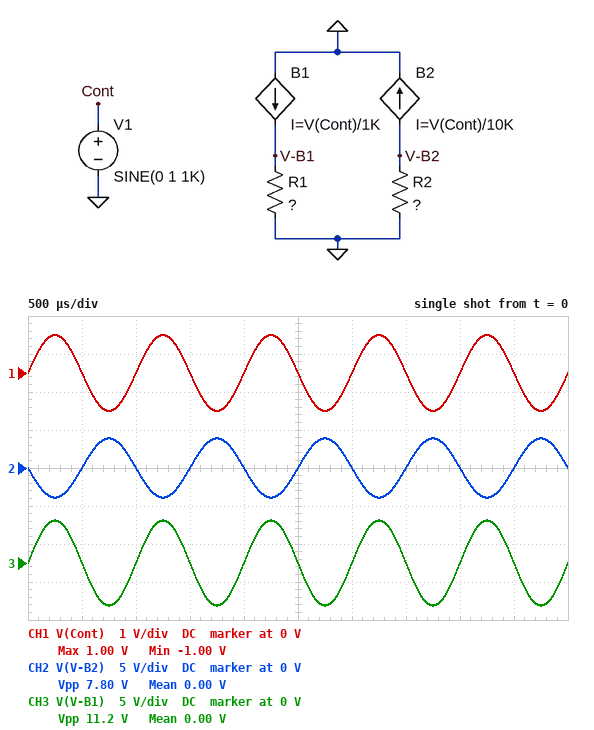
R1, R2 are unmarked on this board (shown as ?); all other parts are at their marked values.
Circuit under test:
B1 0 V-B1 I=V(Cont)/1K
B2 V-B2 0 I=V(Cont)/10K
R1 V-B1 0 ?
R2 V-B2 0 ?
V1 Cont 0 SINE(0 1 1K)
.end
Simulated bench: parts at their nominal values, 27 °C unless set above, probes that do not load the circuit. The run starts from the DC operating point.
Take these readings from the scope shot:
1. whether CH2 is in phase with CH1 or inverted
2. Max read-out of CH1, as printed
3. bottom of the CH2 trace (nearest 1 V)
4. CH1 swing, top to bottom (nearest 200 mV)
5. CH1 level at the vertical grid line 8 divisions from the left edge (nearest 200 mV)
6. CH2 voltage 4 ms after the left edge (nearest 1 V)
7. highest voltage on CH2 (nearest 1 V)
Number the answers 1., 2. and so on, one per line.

1. inverted
2. 1.00 V
3. -4 V
4. 2.0 V
5. 0 V
6. 0 V
7. 4 V
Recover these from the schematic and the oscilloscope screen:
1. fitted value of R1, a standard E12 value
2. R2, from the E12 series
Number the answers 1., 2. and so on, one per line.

1. 5.6 kΩ
2. 39 kΩ
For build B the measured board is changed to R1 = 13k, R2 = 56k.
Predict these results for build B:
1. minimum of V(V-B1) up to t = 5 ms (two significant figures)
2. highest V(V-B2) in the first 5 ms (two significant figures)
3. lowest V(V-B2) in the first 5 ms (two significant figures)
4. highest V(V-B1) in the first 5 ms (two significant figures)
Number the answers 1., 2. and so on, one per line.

1. -13 V
2. 5.6 V
3. -5.6 V
4. 13 V
